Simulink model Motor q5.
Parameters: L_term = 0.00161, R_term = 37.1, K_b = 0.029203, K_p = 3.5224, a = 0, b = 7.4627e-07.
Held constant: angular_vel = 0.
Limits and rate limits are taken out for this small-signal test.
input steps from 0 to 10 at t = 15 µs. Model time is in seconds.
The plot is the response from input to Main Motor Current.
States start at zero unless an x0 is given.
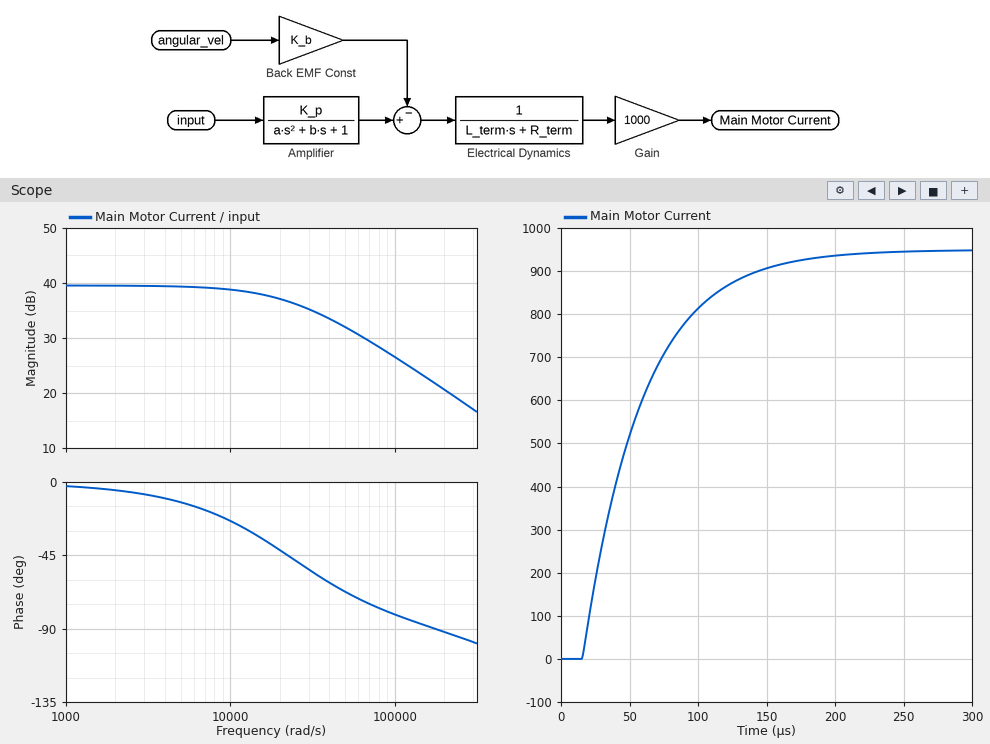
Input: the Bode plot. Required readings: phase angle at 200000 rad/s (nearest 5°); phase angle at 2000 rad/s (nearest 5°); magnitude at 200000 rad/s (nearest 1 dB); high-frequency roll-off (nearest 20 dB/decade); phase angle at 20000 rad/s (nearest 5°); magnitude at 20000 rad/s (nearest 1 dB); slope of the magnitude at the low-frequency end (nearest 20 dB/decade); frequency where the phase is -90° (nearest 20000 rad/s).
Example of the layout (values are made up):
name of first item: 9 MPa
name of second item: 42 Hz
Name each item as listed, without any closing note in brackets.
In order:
phase angle at 200000 rad/s: -90°
phase angle at 2000 rad/s: -5°
magnitude at 200000 rad/s: 21 dB
high-frequency roll-off: -20 dB/decade
phase angle at 20000 rad/s: -40°
magnitude at 20000 rad/s: 37 dB
slope of the magnitude at the low-frequency end: 0 dB/decade
frequency where the phase is -90°: 180000 rad/s
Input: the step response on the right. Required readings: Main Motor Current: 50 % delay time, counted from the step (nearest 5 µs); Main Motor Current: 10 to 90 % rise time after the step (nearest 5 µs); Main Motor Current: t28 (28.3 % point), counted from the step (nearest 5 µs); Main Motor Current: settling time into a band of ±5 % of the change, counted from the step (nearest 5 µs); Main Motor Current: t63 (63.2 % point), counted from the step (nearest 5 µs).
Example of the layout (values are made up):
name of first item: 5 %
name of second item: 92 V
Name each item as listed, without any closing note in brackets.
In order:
Main Motor Current: 50 % delay time, counted from the step: 30 µs
Main Motor Current: 10 to 90 % rise time after the step: 95 µs
Main Motor Current: t28 (28.3 % point), counted from the step: 15 µs
Main Motor Current: settling time into a band of ±5 % of the change, counted from the step: 130 µs
Main Motor Current: t63 (63.2 % point), counted from the step: 45 µs
